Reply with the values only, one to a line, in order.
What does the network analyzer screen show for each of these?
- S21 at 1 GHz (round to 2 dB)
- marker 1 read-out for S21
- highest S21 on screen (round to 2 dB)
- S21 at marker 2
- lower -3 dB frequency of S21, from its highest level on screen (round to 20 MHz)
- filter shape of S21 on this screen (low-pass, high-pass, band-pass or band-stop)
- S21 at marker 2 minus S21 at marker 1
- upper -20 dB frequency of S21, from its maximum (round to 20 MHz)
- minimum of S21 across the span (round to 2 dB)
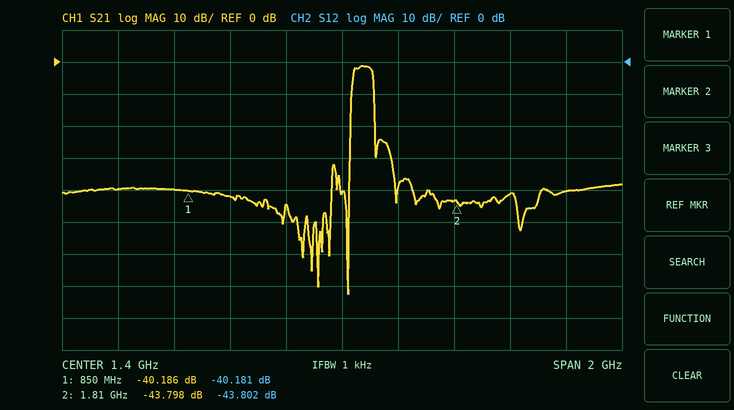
-42 dB
-40.186 dB
-2 dB
-43.798 dB
1.44 GHz
band-pass
-3.612 dB
1.52 GHz
-72 dB
